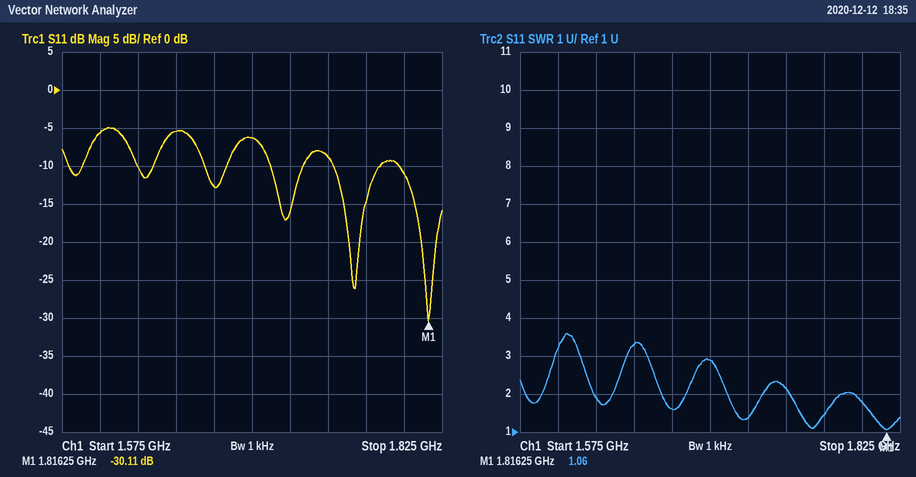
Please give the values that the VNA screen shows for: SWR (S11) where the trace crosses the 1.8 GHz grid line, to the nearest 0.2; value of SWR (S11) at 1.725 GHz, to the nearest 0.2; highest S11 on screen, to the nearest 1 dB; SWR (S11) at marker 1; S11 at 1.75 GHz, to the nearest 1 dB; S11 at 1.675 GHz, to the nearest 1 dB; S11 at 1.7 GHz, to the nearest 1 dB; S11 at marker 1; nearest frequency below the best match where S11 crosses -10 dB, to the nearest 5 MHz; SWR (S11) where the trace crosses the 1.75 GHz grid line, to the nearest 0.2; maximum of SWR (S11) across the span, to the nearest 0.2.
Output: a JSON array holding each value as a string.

["1.8", "1.4", "-5 dB", "1.06", "-9 dB", "-13 dB", "-6 dB", "-30.11 dB", "1.795 GHz", "2.2", "3.6"]
